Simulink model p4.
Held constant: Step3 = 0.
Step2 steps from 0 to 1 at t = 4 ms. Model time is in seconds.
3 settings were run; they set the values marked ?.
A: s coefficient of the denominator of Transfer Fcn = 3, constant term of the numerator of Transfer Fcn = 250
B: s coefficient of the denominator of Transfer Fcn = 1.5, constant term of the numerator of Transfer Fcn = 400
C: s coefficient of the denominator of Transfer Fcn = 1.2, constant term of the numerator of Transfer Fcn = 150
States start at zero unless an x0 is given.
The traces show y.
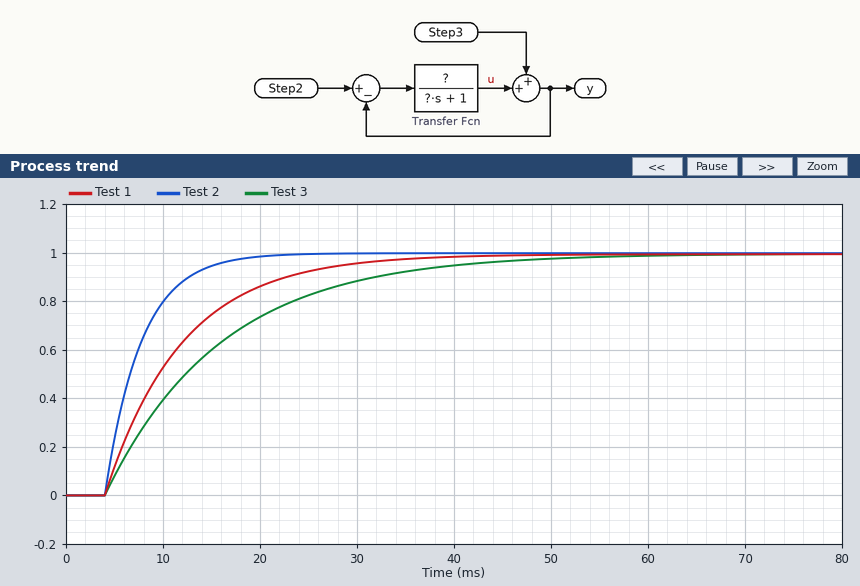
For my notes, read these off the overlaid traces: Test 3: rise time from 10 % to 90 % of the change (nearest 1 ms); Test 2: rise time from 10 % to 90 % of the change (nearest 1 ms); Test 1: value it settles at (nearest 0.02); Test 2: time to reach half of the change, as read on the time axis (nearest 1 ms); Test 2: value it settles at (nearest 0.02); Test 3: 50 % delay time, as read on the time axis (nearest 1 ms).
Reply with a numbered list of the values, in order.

1. 26 ms
2. 8 ms
3. 1.00
4. 7 ms
5. 1.00
6. 12 ms
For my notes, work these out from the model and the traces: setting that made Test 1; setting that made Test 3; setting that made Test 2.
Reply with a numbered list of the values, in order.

1. C
2. A
3. B
